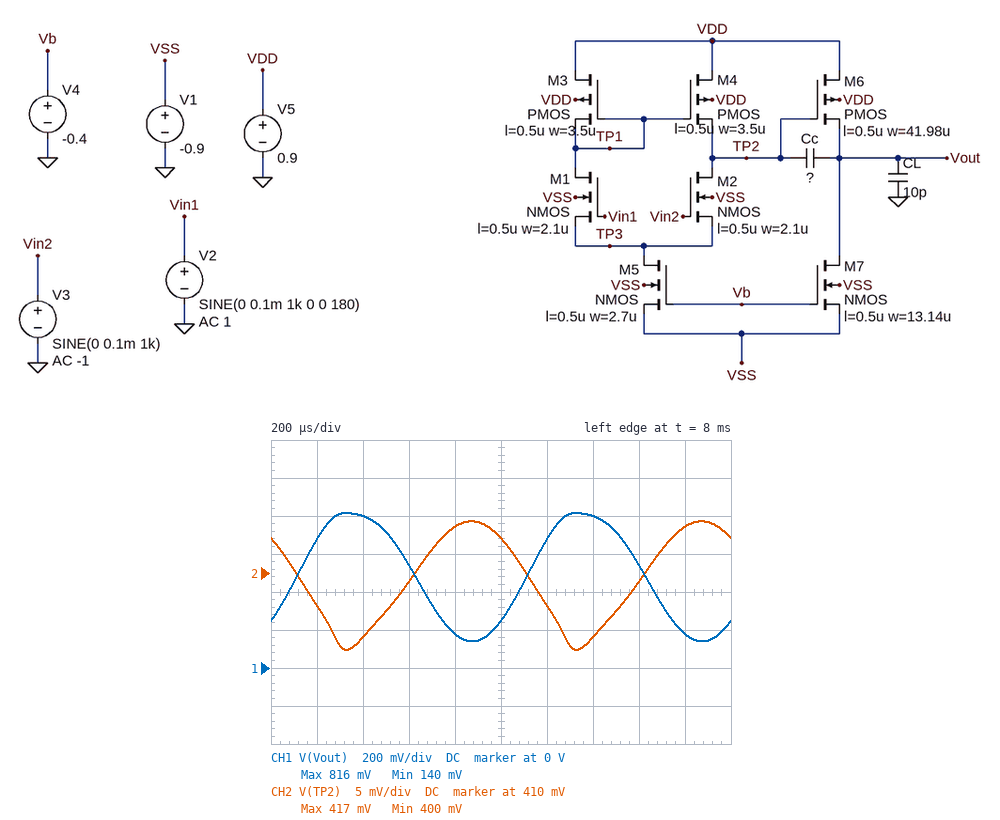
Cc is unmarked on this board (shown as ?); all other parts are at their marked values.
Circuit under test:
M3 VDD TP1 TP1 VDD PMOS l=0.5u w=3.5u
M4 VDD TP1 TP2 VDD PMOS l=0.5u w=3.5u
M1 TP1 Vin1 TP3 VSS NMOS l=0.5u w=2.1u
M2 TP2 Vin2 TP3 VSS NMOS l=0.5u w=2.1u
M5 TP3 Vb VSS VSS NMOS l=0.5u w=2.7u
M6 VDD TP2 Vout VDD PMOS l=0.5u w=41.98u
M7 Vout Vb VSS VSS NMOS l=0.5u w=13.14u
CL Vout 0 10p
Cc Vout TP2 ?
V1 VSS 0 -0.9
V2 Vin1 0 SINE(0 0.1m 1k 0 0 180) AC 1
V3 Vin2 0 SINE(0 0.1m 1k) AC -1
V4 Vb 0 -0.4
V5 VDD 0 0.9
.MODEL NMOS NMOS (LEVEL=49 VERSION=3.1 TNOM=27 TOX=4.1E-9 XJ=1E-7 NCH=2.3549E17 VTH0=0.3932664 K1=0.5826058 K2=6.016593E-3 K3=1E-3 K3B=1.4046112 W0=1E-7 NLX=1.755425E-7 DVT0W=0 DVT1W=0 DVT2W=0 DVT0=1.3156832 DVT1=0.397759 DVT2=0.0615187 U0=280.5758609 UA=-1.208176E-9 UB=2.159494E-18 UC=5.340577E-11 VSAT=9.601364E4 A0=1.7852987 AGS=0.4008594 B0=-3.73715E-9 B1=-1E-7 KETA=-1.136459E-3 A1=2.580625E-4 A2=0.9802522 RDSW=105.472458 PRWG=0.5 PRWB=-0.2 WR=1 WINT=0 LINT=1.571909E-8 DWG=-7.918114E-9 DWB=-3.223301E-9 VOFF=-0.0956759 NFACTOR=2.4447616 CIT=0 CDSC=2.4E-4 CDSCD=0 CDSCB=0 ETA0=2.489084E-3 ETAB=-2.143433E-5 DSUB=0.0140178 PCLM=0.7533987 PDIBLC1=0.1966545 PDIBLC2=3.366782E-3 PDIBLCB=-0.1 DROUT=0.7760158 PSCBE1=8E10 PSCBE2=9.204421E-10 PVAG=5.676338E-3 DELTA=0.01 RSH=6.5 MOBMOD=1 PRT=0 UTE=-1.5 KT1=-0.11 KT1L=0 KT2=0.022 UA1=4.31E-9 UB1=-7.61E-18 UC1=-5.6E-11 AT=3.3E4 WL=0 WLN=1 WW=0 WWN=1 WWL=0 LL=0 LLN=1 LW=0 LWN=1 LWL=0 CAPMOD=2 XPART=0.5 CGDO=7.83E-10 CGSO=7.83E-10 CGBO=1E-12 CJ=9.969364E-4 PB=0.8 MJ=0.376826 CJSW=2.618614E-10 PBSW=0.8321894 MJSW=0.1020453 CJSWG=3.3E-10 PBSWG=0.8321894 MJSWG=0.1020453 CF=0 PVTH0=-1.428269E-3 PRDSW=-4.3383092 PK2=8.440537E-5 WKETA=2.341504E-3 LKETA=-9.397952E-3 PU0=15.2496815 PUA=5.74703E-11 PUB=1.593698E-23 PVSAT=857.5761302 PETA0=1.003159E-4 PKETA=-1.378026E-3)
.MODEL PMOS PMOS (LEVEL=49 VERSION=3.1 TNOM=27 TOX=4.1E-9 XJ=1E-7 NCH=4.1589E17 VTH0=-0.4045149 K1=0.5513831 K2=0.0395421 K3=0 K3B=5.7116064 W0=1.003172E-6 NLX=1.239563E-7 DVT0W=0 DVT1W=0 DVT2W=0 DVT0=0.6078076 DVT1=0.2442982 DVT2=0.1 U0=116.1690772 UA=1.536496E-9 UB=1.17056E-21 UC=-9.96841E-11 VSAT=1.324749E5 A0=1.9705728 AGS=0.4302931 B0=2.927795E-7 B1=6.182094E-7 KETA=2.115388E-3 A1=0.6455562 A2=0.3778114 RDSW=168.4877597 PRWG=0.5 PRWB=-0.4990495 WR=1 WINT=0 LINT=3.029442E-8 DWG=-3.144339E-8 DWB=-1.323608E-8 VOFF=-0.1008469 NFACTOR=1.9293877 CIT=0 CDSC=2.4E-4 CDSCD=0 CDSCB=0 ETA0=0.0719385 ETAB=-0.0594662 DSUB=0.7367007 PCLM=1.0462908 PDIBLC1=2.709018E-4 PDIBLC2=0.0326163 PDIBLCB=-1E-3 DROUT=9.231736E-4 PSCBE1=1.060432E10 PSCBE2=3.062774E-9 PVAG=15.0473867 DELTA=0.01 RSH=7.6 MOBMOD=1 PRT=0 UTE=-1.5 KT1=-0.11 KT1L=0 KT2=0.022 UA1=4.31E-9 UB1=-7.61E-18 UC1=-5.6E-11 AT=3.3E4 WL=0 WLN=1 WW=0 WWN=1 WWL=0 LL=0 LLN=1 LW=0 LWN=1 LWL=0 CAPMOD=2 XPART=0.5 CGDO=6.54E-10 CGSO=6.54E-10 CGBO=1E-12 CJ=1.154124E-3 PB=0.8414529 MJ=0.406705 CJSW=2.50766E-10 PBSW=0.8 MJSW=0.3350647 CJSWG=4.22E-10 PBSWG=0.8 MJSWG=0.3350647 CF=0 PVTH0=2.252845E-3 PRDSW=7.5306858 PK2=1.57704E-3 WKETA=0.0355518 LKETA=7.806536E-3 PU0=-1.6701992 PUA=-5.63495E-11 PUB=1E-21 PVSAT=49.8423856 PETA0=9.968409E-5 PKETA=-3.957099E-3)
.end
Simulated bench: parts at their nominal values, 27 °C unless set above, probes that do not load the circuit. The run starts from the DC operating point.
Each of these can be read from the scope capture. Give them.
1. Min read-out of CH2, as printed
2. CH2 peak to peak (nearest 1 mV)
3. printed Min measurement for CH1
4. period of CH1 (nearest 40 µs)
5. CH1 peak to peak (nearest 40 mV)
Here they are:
400 mV
17 mV
140 mV
1.00 ms
680 mV
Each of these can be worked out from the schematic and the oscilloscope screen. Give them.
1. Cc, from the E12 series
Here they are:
1.2 pF
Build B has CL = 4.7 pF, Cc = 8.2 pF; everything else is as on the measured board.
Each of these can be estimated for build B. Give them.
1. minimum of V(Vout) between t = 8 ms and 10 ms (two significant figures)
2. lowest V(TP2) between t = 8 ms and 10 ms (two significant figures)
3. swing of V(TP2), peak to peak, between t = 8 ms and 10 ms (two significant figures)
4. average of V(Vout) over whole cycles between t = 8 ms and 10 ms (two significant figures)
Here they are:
440 mV
410 mV
3.2 mV
520 mV
